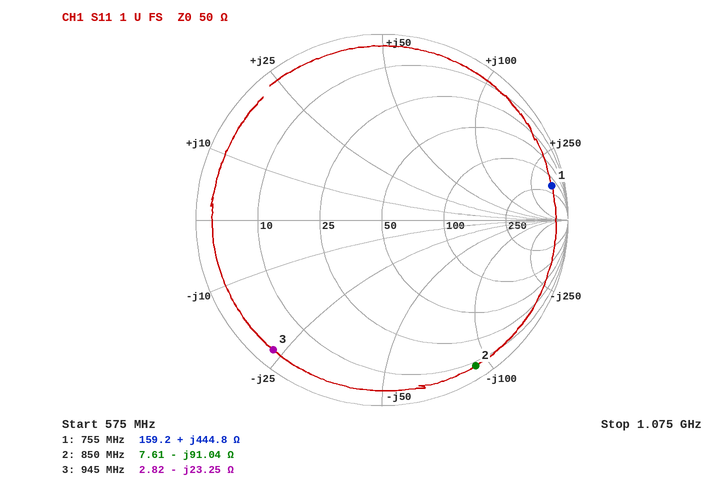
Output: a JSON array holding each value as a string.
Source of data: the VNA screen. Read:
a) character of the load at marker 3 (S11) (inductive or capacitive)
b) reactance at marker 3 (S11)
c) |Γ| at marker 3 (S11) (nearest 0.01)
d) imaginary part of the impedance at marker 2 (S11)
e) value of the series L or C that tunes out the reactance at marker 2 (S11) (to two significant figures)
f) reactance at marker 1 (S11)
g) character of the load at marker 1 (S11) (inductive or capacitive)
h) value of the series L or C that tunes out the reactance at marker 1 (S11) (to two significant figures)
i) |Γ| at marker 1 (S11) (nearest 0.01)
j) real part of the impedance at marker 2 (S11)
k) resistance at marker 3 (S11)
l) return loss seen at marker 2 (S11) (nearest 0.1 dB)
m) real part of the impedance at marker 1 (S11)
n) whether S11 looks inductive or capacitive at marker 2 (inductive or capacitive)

["capacitive", "-23.25 Ω", "0.91", "-91.04 Ω", "17 nH", "+444.8 Ω", "inductive", "470 fF", "0.93", "7.61 Ω", "2.82 Ω", "0.6 dB", "159.2 Ω", "capacitive"]
